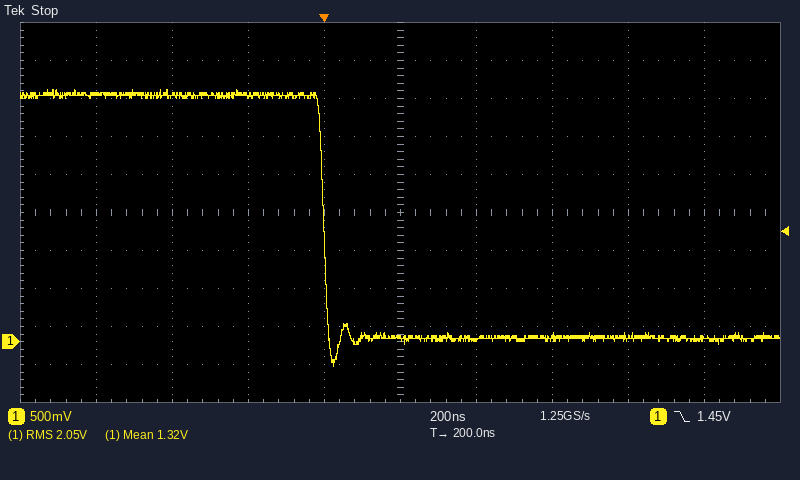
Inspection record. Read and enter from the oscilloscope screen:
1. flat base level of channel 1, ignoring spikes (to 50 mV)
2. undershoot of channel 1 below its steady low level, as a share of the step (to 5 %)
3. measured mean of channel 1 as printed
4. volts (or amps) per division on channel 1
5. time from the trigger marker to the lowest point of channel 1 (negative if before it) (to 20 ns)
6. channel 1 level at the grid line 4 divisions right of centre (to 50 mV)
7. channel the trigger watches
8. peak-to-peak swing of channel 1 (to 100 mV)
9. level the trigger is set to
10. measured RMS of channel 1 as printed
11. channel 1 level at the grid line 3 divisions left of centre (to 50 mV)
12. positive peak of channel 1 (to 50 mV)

50 mV
10 %
1.32 V
500 mV
+20 ns
50 mV
channel 1
3.60 V
1.45 V
2.05 V
3.25 V
3.30 V
